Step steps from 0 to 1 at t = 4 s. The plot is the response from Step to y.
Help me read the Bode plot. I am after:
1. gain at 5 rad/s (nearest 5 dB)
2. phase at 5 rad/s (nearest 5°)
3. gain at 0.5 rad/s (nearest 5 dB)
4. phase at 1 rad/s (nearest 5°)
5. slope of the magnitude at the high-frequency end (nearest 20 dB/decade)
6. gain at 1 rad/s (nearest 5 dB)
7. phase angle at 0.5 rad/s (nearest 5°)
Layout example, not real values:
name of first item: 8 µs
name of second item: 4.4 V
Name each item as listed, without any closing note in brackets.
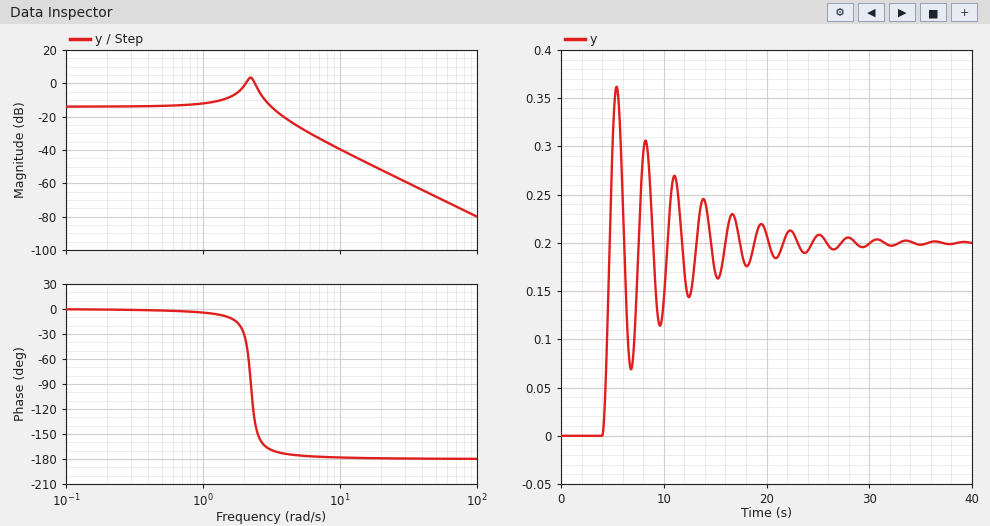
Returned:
gain at 5 rad/s: -25 dB
phase at 5 rad/s: -175°
gain at 0.5 rad/s: -15 dB
phase at 1 rad/s: -5°
slope of the magnitude at the high-frequency end: -40 dB/decade
gain at 1 rad/s: -10 dB
phase angle at 0.5 rad/s: 0°
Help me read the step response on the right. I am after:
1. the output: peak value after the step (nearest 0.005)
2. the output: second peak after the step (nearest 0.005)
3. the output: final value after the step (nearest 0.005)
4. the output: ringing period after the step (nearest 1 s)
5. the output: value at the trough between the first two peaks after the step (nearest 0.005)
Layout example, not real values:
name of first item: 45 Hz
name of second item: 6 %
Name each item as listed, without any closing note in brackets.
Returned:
the output: peak value after the step: 0.360
the output: second peak after the step: 0.305
the output: final value after the step: 0.200
the output: ringing period after the step: 3 s
the output: value at the trough between the first two peaks after the step: 0.070
